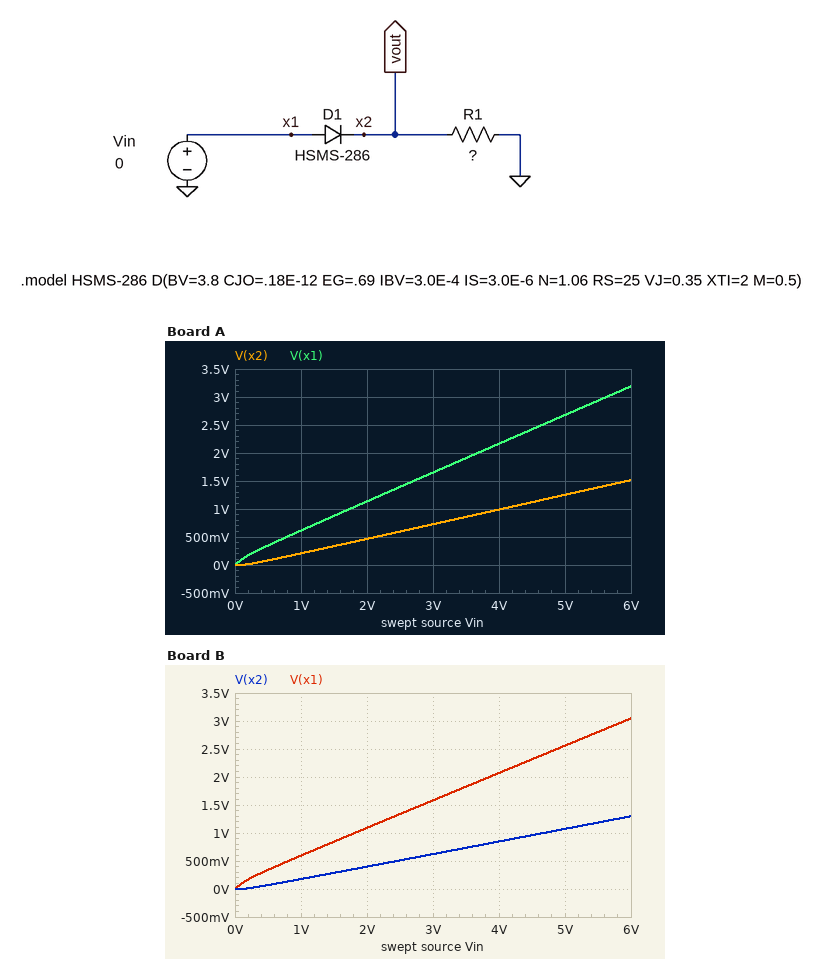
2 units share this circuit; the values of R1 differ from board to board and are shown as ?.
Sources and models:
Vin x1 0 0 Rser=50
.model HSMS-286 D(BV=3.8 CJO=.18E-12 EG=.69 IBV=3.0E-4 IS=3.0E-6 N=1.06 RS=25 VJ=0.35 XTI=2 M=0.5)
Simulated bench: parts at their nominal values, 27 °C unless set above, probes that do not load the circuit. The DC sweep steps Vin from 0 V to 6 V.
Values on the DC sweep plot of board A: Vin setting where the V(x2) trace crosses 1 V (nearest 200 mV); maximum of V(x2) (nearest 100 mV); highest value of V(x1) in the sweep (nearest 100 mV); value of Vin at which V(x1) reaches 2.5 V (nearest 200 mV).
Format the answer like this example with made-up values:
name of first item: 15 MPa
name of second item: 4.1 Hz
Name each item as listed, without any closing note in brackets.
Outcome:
Vin setting where the V(x2) trace crosses 1 V: 4.0 V
maximum of V(x2): 1.5 V
highest value of V(x1) in the sweep: 3.2 V
value of Vin at which V(x1) reaches 2.5 V: 4.6 V
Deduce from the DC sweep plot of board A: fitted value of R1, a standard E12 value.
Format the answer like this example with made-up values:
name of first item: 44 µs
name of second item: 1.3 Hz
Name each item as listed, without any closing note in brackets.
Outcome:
fitted value of R1, a standard E12 value: 27 Ω
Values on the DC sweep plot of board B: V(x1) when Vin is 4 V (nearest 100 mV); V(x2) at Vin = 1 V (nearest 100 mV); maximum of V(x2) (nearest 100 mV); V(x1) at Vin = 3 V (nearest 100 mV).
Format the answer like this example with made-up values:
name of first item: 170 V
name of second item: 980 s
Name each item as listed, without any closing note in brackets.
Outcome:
V(x1) when Vin is 4 V: 2.1 V
V(x2) at Vin = 1 V: 200 mV
maximum of V(x2): 1.3 V
V(x1) at Vin = 3 V: 1.6 V
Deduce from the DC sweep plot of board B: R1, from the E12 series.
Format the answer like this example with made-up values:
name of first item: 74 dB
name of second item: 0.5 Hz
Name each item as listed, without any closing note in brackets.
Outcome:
R1, from the E12 series: 22 Ω
